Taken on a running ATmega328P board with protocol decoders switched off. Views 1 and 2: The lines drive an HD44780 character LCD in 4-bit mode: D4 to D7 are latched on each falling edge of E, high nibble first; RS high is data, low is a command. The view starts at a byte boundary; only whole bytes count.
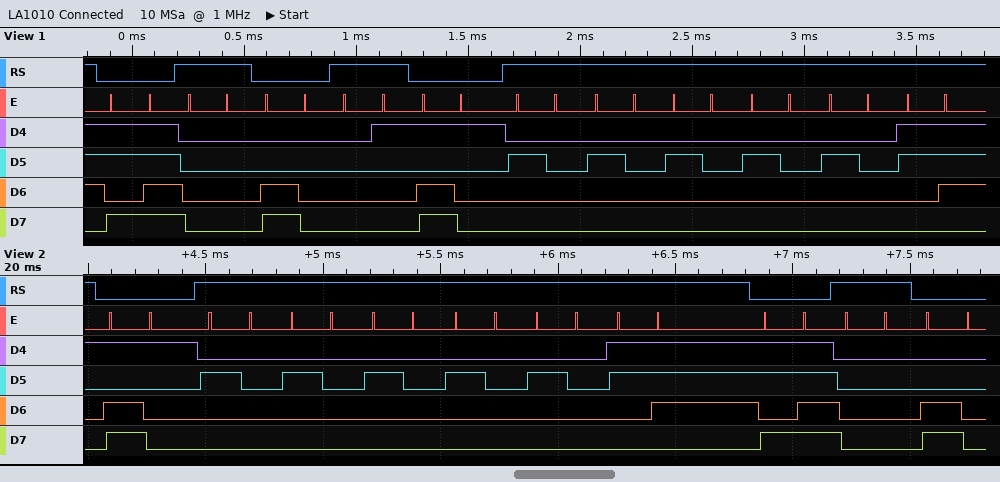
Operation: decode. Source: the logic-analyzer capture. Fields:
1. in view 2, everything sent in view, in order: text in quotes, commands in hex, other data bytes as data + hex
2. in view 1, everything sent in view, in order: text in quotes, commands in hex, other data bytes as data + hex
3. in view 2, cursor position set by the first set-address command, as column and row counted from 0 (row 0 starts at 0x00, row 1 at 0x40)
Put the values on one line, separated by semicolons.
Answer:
0xD1 "     7" 0xBF data 00 0xC0; 0xBF data 00 0xC0 data 01 0xD1 "     7"; column 17, row 1
